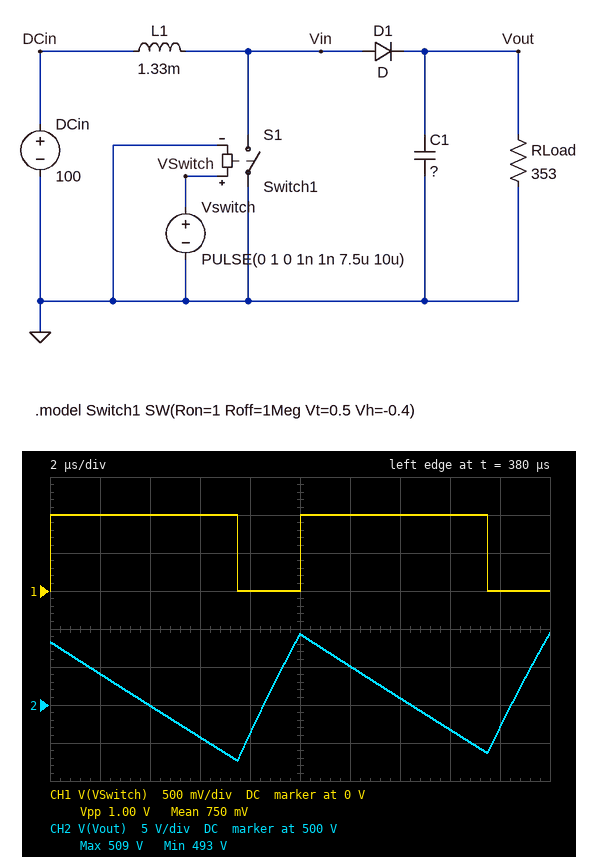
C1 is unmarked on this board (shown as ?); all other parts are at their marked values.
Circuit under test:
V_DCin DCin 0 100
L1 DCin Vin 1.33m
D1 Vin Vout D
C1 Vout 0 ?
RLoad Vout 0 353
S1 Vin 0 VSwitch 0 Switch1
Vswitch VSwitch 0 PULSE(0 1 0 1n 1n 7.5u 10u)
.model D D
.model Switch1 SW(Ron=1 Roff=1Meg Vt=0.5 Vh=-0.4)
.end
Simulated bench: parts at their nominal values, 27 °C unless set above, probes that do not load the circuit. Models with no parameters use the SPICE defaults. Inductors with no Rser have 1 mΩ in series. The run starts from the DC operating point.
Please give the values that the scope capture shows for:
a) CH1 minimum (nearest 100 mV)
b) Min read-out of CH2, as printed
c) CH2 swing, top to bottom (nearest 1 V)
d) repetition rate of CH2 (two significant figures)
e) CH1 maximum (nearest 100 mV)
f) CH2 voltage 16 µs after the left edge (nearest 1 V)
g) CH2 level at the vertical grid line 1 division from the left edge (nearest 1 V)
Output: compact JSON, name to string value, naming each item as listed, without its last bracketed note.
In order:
{"CH1 minimum": "0 V", "Min read-out of CH2, as printed": "493 V", "CH2 swing, top to bottom": "17 V", "repetition rate of CH2": "100 kHz", "CH1 maximum": "1.0 V", "CH2 voltage 16 µs after the left edge": "497 V", "CH2 level at the vertical grid line 1 division from the left edge": "504 V"}
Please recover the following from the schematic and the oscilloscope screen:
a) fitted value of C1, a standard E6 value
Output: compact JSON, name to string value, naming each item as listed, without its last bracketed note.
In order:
{"fitted value of C1, a standard E6 value": "680 nF"}
